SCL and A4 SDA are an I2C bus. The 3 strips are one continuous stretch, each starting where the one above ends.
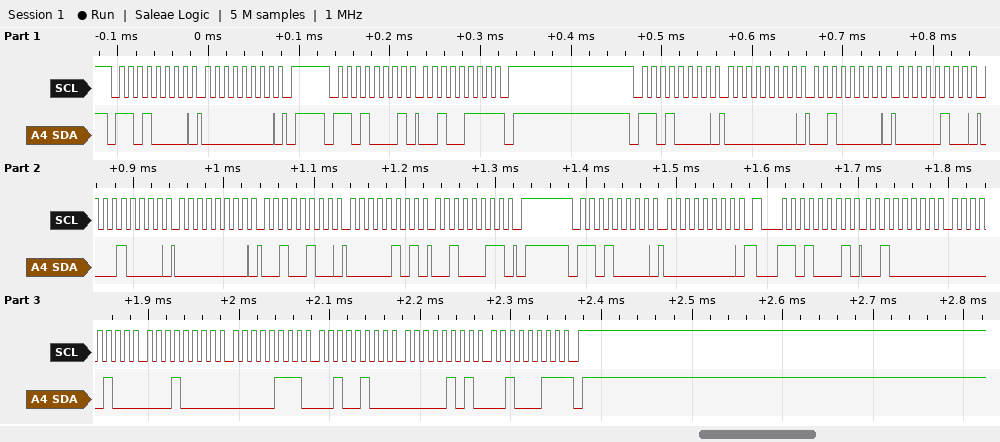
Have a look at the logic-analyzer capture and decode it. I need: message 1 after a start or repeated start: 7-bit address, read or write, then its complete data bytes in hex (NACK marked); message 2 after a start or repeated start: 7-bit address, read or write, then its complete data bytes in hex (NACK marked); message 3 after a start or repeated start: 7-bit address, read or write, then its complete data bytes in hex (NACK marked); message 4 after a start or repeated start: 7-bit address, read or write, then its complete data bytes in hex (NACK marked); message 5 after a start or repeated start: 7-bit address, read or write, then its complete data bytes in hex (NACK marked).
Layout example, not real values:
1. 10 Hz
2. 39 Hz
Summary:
1. 0x68 write: 00
2. 0x68 read: 27 NACK
3. 0x68 write: 00 20 04 10 00 24 05 23
4. 0x68 write: 00
5. 0x68 read: 20 04 10 07 24 05 23 NACK
